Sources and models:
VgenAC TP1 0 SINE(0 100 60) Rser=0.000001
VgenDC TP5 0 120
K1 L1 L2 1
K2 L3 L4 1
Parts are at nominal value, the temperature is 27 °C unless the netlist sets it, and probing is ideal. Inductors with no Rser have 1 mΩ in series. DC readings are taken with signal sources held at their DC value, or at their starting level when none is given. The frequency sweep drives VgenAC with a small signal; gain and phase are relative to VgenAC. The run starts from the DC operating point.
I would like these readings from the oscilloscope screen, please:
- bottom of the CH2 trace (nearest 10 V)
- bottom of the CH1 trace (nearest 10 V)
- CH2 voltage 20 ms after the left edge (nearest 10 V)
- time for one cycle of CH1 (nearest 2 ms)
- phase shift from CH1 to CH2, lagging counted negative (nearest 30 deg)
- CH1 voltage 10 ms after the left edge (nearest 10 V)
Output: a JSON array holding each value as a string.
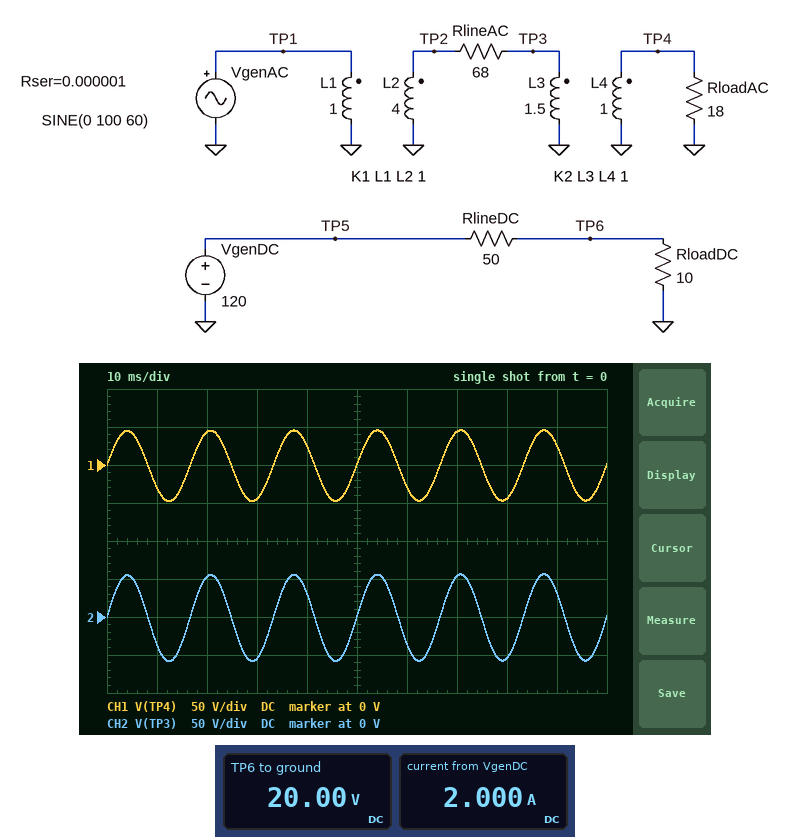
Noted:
["-60 V", "-50 V", "50 V", "16 ms", "0 deg", "-30 V"]
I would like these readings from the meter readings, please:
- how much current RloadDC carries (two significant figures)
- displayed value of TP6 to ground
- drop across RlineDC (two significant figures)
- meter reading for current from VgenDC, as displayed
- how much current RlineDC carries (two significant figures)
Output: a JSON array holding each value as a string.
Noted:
["2.0 A", "20.00 V", "100 V", "2.000 A", "2.0 A"]
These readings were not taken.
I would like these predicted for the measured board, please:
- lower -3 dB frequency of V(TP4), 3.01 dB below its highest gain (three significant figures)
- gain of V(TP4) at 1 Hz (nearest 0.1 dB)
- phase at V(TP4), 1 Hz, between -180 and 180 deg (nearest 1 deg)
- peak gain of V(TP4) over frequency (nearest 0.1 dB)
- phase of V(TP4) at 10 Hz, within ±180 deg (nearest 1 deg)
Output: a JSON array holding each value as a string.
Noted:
["2.05 Hz", "-13.8 dB", "64 deg", "-6.7 dB", "12 deg"]
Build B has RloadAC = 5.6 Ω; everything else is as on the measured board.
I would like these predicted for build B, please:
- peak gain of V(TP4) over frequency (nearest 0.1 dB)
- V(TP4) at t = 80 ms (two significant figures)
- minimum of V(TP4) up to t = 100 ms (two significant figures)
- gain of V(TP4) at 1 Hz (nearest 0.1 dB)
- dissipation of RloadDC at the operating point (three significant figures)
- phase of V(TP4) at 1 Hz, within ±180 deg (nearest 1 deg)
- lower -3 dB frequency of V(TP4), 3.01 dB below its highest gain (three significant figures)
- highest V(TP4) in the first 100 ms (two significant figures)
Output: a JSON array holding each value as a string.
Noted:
["-14.9 dB", "-17 V", "-18 V", "-17.0 dB", "40.0 W", "38 deg", "793 mHz", "18 V"]
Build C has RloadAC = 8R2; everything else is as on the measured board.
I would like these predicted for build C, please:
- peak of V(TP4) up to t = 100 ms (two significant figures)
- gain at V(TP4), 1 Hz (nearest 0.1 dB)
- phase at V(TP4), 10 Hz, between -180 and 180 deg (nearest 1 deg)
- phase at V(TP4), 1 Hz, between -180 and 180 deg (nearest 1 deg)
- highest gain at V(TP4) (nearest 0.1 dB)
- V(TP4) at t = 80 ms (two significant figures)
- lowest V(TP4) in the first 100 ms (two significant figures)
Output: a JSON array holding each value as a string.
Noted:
["25 V", "-15.5 dB", "6 deg", "48 deg", "-12.0 dB", "-24 V", "-25 V"]
